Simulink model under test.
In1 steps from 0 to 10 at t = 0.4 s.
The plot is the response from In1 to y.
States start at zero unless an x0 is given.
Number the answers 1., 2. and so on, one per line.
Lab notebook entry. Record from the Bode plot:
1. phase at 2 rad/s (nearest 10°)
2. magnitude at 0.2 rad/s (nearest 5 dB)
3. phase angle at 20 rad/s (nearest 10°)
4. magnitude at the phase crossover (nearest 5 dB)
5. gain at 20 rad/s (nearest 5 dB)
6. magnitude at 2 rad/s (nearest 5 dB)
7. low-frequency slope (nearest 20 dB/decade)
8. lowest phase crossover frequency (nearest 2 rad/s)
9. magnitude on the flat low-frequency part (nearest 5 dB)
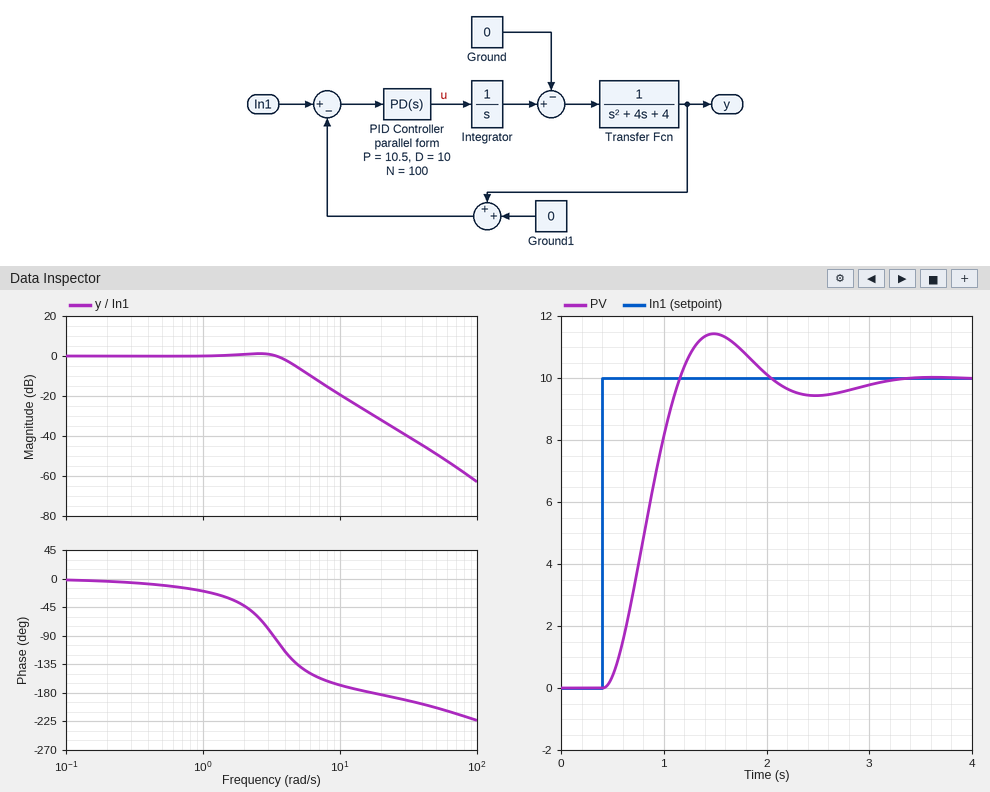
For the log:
1. -40°
2. 0 dB
3. -180°
4. -30 dB
5. -30 dB
6. 0 dB
7. 0 dB/decade
8. 18 rad/s
9. 0 dB
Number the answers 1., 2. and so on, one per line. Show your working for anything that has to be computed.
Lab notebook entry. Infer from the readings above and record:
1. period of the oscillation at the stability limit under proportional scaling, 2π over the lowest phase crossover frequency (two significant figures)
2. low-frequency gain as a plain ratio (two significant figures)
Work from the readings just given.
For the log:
1. 2π / 18 = 0.35 s
2. 10^(0 / 20) = 1.0
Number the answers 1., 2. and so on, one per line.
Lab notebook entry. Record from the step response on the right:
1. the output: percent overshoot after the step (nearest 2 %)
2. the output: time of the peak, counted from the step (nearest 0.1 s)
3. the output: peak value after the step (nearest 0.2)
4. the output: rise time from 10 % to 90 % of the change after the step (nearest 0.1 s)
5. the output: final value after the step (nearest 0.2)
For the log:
1. 14 %
2. 1.1 s
3. 11.4
4. 0.5 s
5. 10.0
